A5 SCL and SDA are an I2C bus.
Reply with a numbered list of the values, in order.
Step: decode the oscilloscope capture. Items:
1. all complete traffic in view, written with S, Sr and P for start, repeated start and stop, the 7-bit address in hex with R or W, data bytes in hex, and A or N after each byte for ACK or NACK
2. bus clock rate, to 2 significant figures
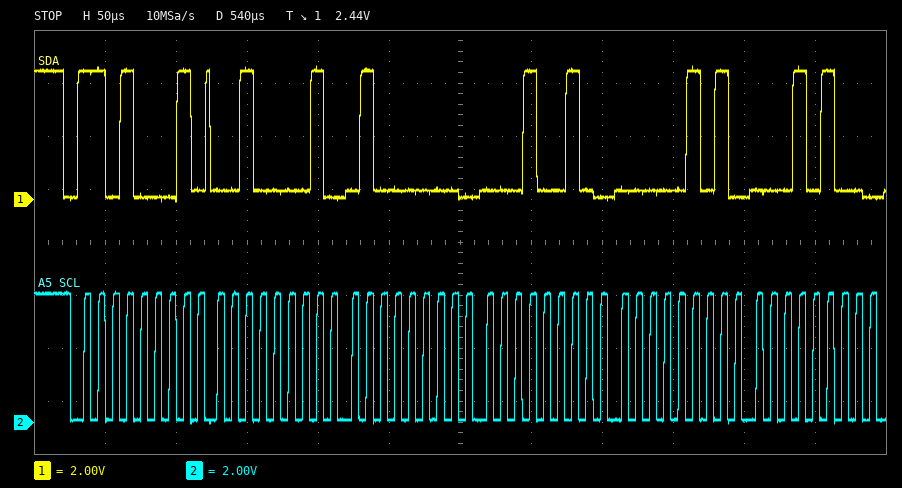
1. S 68R A 21 A 40 A 12 A 05 A 14 A
2. 100 kHz
